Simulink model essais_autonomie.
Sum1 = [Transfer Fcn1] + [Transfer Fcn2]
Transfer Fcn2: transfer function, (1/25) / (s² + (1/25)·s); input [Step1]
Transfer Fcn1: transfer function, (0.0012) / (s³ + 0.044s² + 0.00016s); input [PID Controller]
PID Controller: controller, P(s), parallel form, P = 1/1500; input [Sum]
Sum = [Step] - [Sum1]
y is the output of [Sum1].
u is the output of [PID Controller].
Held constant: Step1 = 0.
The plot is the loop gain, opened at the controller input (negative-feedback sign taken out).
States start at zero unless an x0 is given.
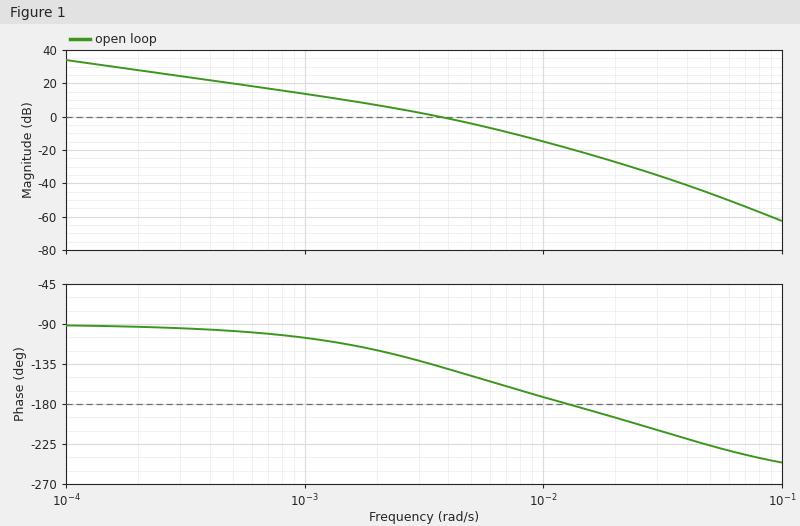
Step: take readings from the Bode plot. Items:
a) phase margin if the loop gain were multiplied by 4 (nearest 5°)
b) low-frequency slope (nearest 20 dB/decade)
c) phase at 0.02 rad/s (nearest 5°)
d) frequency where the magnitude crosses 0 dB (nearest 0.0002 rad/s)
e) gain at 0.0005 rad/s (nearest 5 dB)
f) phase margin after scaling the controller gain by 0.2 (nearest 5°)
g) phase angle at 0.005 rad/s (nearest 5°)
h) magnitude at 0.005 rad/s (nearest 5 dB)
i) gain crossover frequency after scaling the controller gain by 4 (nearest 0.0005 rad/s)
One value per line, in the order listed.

15°
-20 dB/decade
-195°
0.0036 rad/s
20 dB
75°
-150°
-5 dB
0.0085 rad/s
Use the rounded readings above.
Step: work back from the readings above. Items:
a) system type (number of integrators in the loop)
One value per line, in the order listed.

1
